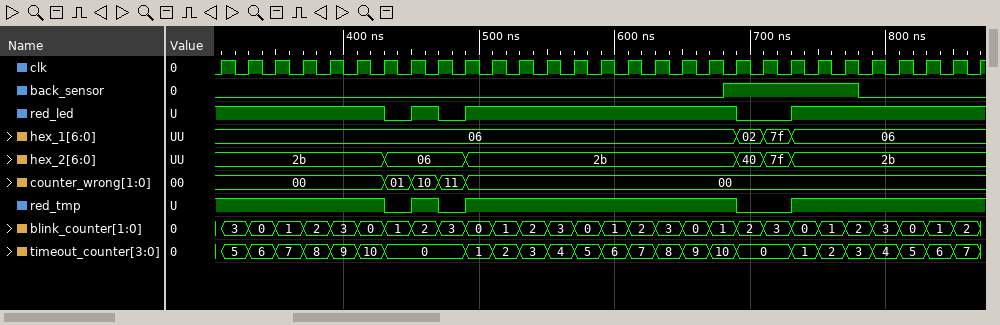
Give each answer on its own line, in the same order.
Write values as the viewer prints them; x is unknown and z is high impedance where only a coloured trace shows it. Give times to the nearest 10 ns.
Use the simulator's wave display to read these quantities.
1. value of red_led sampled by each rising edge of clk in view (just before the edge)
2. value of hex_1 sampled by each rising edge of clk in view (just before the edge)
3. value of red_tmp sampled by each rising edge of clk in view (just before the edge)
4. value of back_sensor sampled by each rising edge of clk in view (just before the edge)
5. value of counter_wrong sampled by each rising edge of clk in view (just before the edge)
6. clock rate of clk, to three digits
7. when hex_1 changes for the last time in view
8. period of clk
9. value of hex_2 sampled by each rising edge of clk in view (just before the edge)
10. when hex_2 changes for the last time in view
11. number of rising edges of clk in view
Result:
1 1 1 1 1 1 1 0 1 0 1 1 1 1 1 1 1 1 1 1 0 0 1 1 1 1 1 1 1
06, 06, 06, 06, 06, 06, 06, 06, 06, 06, 06, 06, 06, 06, 06, 06, 06, 06, 06, 06, 02, 7f, 06, 06, 06, 06, 06, 06, 06
1 1 1 1 1 1 1 0 1 0 1 1 1 1 1 1 1 1 1 1 0 0 1 1 1 1 1 1 1
0 0 0 0 0 0 0 0 0 0 0 0 0 0 0 0 0 0 0 1 1 1 1 1 0 0 0 0 0
00, 00, 00, 00, 00, 00, 00, 01, 10, 11, 00, 00, 00, 00, 00, 00, 00, 00, 00, 00, 00, 00, 00, 00, 00, 00, 00, 00, 00
50.0 MHz
730 ns
20 ns
2b, 2b, 2b, 2b, 2b, 2b, 2b, 06, 06, 06, 2b, 2b, 2b, 2b, 2b, 2b, 2b, 2b, 2b, 2b, 40, 7f, 2b, 2b, 2b, 2b, 2b, 2b, 2b
730 ns
29
